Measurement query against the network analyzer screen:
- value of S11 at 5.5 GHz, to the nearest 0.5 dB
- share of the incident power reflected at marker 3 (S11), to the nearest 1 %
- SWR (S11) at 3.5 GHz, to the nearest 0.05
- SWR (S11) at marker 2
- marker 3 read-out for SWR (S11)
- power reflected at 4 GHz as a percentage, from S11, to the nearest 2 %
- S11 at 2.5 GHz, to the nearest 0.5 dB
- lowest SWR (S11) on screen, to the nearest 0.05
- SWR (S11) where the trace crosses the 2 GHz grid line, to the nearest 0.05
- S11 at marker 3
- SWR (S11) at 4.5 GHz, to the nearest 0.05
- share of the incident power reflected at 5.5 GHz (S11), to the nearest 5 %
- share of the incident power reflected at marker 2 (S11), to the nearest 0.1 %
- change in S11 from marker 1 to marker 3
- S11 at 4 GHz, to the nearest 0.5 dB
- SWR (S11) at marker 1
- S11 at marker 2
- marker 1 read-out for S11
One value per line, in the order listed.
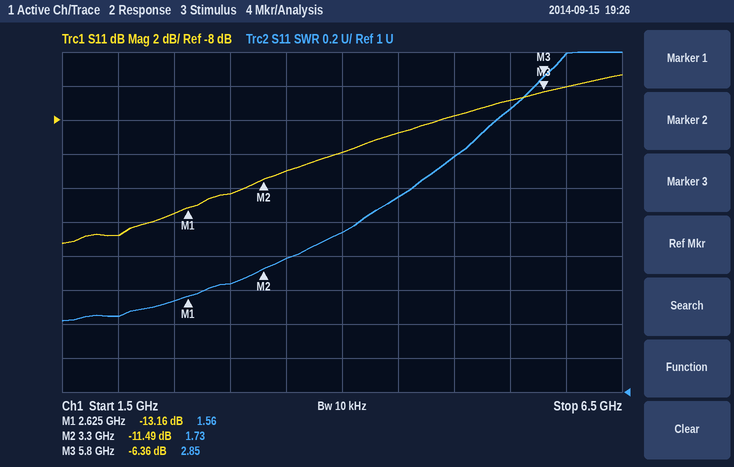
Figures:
-7.0 dB
23 %
1.80
1.73
2.85
10 %
-13.5 dB
1.40
1.45
-6.36 dB
2.15
20 %
7.1 %
6.80 dB
-10.0 dB
1.56
-11.49 dB
-13.16 dB
